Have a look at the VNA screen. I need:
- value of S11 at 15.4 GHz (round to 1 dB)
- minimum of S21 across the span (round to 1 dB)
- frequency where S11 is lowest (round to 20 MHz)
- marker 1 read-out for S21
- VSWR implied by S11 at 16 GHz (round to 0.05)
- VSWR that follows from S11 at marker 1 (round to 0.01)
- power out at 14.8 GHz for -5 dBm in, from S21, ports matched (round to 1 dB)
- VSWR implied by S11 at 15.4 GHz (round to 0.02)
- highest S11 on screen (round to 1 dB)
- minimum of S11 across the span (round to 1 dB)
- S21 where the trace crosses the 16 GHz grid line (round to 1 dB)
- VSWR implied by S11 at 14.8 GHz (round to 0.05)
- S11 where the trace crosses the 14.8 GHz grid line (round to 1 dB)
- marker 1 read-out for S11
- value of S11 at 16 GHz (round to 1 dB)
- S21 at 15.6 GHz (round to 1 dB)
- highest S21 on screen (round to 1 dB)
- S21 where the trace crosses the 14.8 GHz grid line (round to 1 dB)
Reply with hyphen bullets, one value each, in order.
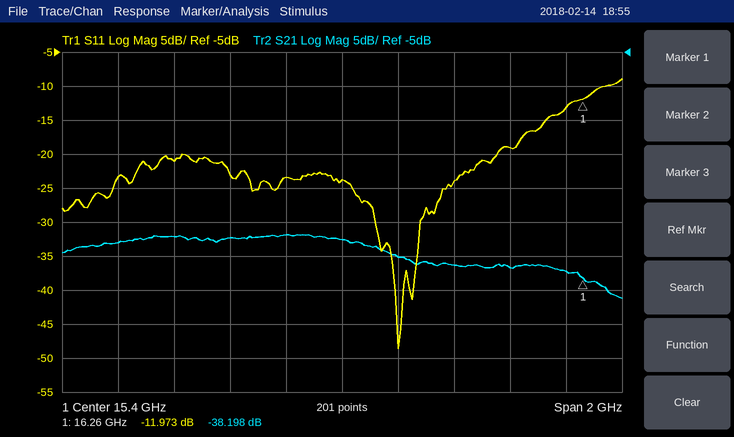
- -24 dB
- -41 dB
- 15.60 GHz
- -38.198 dB
- 1.25
- 1.67
- -37 dBm
- 1.14
- -9 dB
- -49 dB
- -37 dB
- 1.20
- -21 dB
- -11.973 dB
- -19 dB
- -35 dB
- -32 dB
- -32 dB
